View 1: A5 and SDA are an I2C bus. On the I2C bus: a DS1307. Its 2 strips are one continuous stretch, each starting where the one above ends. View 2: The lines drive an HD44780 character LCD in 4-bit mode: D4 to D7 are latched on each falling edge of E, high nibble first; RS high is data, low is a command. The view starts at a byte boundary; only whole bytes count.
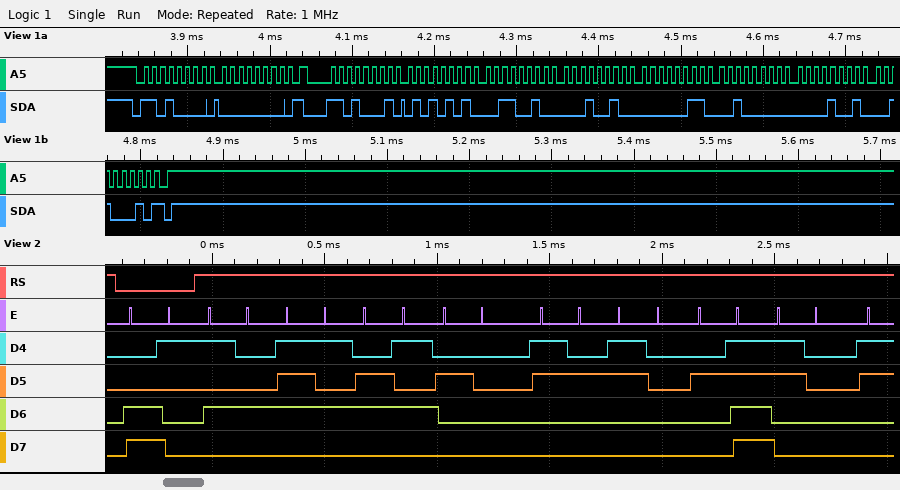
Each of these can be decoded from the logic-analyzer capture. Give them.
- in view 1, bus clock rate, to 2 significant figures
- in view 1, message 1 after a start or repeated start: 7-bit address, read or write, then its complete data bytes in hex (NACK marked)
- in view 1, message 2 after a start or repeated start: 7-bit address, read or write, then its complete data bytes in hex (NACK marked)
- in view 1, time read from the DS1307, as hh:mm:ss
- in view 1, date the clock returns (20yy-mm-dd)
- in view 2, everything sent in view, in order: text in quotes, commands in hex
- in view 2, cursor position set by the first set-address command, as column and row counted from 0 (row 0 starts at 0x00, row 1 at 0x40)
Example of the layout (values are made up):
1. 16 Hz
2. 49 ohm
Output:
1. 100 kHz
2. 0x68 write: 00
3. 0x68 read: 55 32 12 03 20 09 22 NACK
4. 12:32:55
5. 2022-09-20
6. 0xC1 "Tue 20/0"
7. column 1, row 1
